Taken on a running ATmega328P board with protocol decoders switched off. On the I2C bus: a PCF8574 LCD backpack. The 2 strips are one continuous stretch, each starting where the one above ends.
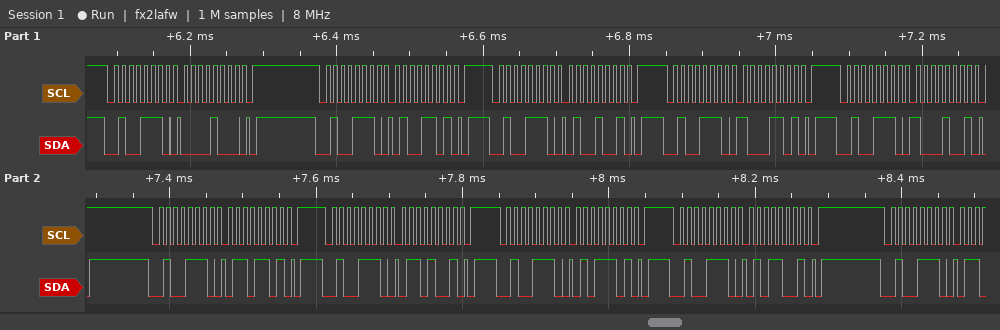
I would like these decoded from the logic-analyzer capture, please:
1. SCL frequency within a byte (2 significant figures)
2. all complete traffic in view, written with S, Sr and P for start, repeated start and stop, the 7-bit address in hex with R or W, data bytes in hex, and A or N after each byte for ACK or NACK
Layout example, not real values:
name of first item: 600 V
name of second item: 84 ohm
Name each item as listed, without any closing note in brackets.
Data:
SCL frequency within a byte: 100 kHz
all complete traffic in view, written with S, Sr and P for start, repeated start and stop, the 7-bit address in hex with R or W, data bytes in hex, and A or N after each byte for ACK or NACK: S 27W A 08 A P S 27W A 4D A P S 27W A 49 A P S 27W A 8D A P S 27W A 89 A P S 27W A 6D A P S 27W A 69 A P S 27W A 5D A P S 27W A 59 A P S 27W A
